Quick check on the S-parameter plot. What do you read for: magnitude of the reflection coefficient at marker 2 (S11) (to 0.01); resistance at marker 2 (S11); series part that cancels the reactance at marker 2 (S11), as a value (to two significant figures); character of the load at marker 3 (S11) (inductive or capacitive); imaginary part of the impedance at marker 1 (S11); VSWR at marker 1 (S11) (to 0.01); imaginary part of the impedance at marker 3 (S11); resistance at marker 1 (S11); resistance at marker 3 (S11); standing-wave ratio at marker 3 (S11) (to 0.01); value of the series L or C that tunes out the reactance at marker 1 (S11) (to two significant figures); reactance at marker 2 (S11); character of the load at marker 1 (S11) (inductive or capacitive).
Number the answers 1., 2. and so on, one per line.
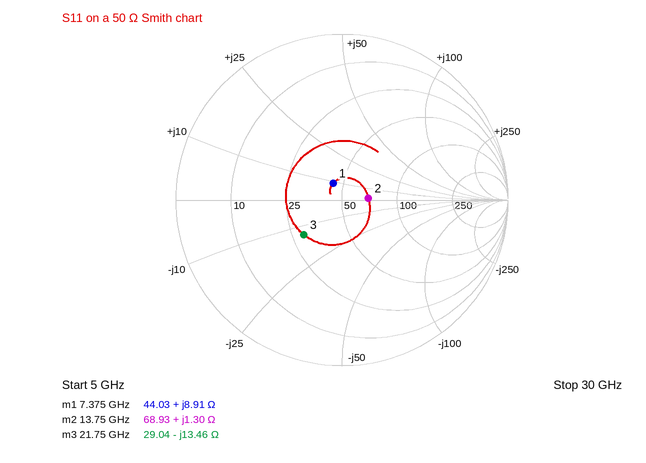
1. 0.16
2. 68.93 Ω
3. 8.9 pF
4. capacitive
5. +8.91 Ω
6. 1.26
7. -13.46 Ω
8. 44.03 Ω
9. 29.04 Ω
10. 1.90
11. 2.4 pF
12. +1.30 Ω
13. inductive
